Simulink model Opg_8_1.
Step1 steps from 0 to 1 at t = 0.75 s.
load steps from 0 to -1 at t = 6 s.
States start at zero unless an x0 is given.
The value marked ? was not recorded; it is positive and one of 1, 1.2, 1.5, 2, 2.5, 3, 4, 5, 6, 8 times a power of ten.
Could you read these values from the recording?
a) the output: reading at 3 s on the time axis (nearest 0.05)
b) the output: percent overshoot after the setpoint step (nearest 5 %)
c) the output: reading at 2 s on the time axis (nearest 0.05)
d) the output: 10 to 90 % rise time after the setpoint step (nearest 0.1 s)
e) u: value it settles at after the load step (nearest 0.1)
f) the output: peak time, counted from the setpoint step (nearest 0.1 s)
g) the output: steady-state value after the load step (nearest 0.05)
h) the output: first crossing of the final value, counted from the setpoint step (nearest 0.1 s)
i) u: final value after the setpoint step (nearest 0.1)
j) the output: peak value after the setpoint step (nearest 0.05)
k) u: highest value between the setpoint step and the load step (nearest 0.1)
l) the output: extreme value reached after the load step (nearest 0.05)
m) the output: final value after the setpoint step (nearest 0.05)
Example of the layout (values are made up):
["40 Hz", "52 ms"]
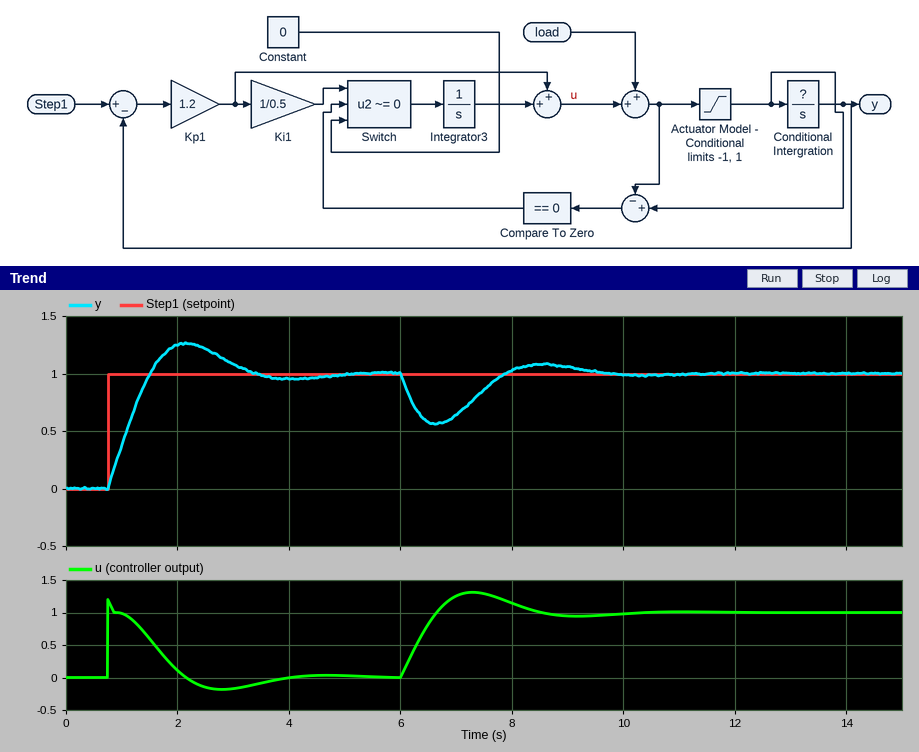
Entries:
["1.10", "25 %", "1.25", "0.6 s", "1.0", "1.4 s", "1.00", "0.8 s", "0.0", "1.25", "1.2", "0.55", "1.00"]
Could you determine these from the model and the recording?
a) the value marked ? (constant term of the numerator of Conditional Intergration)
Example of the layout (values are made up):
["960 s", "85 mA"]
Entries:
["1.5"]
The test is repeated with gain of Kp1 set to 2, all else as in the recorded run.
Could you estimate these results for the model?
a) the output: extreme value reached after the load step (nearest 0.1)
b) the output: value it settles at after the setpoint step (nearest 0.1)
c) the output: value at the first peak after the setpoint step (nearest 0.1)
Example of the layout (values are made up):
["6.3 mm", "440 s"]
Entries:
["0.7", "1.0", "1.1"]
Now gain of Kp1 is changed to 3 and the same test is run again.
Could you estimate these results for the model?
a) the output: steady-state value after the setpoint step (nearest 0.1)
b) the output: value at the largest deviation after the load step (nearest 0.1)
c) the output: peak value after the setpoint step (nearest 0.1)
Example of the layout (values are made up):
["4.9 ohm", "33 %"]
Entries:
["1.0", "0.8", "1.1"]
